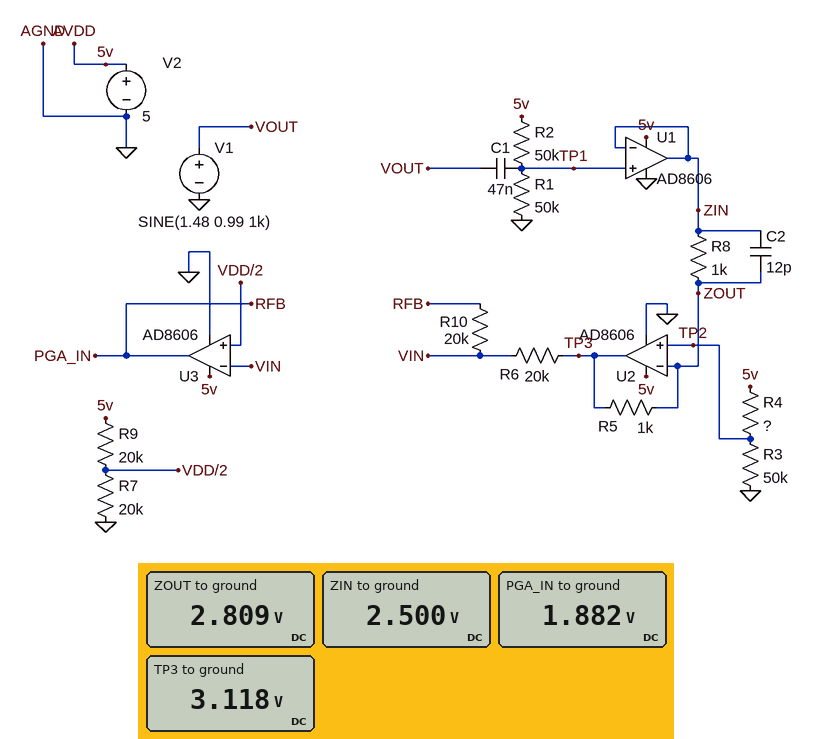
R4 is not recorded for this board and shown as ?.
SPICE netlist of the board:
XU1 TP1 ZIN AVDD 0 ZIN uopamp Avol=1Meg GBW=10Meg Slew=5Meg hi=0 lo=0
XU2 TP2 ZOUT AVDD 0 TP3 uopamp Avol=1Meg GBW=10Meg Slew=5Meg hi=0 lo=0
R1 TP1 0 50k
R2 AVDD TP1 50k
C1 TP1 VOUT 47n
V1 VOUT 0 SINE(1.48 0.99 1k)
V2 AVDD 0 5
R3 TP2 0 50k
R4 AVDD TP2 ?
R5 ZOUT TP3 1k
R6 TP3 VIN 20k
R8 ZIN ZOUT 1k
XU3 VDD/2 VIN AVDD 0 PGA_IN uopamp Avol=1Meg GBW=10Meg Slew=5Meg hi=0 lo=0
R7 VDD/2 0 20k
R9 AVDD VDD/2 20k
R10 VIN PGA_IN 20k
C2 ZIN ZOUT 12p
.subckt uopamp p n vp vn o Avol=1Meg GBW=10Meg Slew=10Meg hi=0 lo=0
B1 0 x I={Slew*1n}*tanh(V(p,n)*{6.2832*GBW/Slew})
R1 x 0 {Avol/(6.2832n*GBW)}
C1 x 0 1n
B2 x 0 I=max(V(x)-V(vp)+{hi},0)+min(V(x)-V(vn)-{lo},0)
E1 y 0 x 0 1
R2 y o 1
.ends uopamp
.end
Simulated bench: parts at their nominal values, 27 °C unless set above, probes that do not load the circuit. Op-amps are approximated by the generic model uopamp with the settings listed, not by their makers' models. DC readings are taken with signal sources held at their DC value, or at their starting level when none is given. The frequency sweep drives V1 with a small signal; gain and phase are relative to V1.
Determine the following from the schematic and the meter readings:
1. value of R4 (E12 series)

39 kΩ
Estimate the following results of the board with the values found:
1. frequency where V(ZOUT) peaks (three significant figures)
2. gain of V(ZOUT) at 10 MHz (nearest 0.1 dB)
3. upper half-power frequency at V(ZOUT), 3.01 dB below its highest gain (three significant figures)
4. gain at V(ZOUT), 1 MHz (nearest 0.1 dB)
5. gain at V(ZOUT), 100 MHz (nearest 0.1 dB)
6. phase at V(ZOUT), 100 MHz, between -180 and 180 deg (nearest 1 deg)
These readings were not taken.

9.60 MHz
-7.1 dB
25.9 MHz
-20.1 dB
-20.2 dB
-77 deg
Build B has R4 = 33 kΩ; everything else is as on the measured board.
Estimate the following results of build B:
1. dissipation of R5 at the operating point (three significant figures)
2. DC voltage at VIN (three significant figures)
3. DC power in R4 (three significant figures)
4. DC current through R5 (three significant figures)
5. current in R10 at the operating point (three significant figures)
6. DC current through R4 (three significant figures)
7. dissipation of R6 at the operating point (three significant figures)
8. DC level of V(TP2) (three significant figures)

262 µW
2.50 V
120 µW
512 µA
51.2 µA
60.2 µA
52.4 µW
3.01 V
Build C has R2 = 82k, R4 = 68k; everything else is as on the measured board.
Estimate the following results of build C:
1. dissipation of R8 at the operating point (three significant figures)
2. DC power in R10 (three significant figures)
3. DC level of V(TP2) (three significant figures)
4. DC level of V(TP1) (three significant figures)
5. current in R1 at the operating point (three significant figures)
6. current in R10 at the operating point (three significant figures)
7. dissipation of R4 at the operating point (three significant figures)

50.5 µW
1.23 µW
2.12 V
1.89 V
37.9 µA
7.83 µA
122 µW
